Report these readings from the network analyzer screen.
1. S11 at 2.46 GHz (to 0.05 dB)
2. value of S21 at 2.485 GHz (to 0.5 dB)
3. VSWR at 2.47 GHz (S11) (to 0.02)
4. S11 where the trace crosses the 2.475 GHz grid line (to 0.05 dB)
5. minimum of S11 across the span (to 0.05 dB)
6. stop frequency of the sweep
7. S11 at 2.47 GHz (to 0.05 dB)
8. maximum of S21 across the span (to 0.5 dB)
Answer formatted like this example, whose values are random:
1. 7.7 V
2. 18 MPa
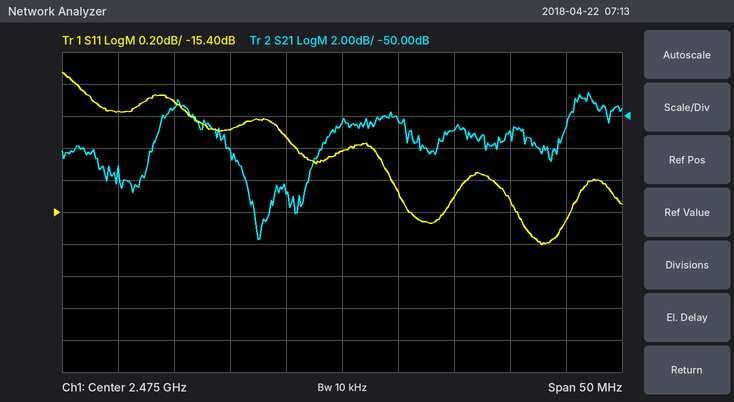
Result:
1. -14.70 dB
2. -51.0 dB
3. 1.44
4. -15.00 dB
5. -15.60 dB
6. 2.5 GHz
7. -14.95 dB
8. -48.5 dB
